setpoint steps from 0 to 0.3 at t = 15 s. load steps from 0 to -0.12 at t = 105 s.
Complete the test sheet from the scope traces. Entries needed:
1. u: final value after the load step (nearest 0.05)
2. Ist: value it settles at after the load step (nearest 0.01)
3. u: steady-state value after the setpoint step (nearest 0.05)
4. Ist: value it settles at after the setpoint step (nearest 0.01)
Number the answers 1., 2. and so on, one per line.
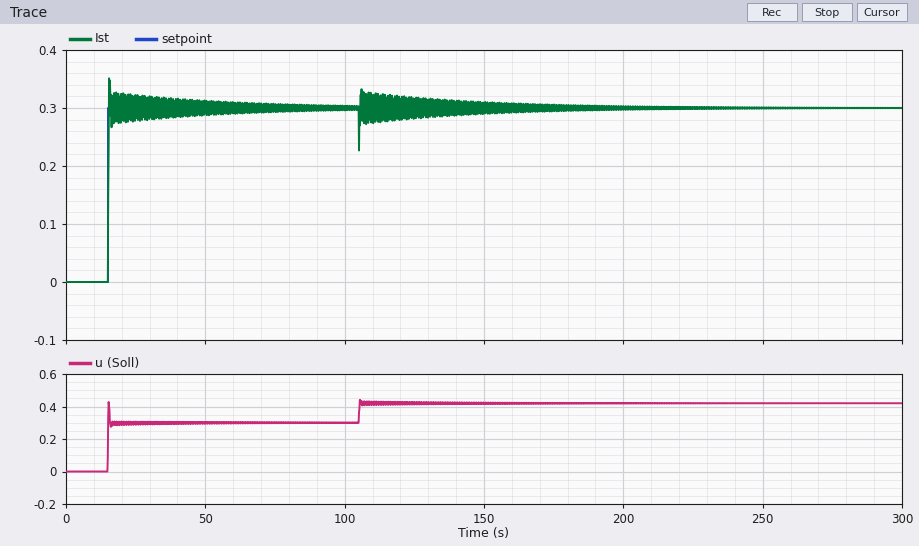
1. 0.40
2. 0.30
3. 0.30
4. 0.30
